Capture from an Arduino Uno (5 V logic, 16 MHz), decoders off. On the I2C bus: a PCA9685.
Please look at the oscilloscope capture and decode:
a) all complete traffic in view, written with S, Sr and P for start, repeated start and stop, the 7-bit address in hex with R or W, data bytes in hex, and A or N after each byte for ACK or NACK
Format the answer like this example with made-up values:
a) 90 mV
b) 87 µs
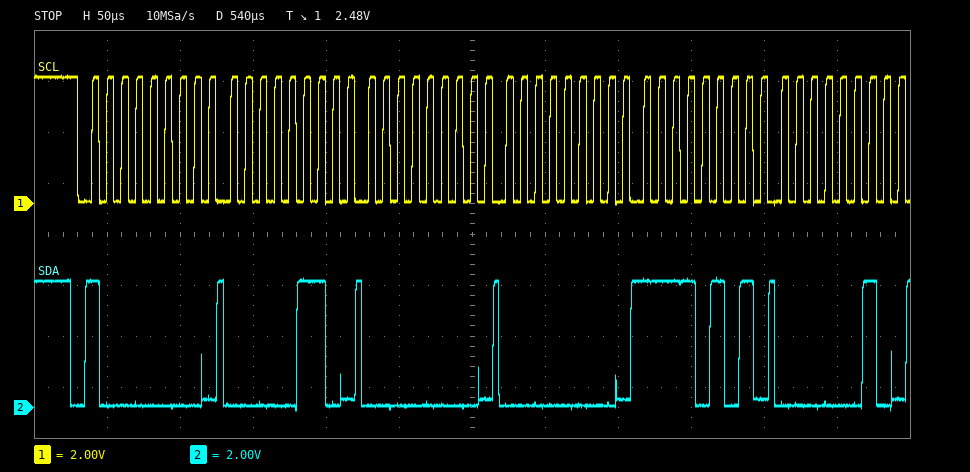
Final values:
a) S 40W A 06 A 00 A 00 A F5 A 02 A
